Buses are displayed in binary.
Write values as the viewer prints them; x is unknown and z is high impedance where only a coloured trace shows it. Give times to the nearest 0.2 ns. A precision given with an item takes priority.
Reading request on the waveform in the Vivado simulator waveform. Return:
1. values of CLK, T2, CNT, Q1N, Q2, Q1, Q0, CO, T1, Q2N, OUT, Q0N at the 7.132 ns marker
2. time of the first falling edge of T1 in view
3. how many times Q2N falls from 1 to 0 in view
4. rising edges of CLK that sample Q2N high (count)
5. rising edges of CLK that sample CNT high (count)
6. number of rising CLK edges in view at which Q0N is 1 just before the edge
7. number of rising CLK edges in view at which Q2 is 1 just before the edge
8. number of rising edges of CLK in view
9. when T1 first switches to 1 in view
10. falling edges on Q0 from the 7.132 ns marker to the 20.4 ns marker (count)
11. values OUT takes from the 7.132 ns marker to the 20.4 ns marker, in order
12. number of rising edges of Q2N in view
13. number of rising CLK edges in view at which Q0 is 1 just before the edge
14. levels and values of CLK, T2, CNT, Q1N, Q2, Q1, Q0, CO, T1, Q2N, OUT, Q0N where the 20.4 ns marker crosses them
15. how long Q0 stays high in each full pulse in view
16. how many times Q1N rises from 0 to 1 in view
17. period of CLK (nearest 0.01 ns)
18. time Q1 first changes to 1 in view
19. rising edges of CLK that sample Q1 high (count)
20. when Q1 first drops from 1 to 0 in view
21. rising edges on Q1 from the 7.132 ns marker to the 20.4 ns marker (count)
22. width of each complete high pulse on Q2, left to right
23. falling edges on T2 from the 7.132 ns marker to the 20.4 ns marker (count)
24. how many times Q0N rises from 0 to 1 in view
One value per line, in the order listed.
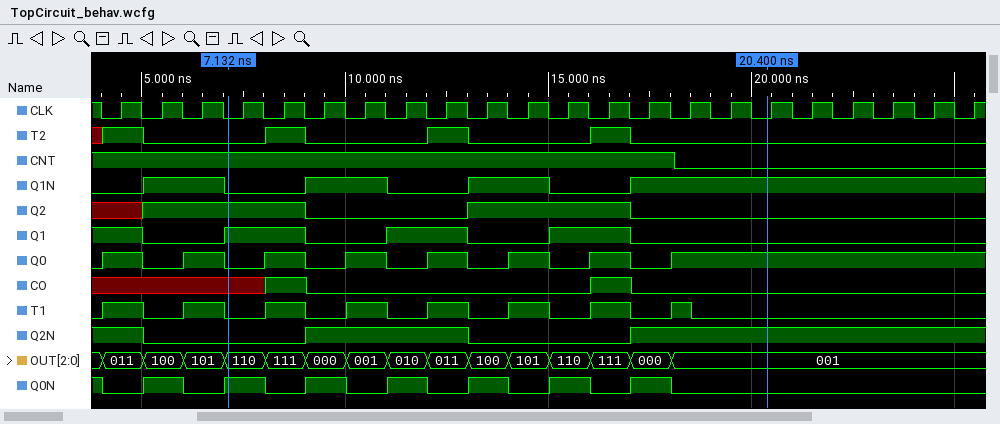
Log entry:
CLK=0, T2=0, CNT=1, Q1N=0, Q2=1, Q1=1, Q0=0, CO=x, T1=0, Q2N=0, OUT=110, Q0N=1
5 ns
2
14
14
7
8
22
4 ns
5
110, 111, 000, 001, 010, 011, 100, 101, 110, 111, 000, 001
2
15
CLK=0, T2=0, CNT=0, Q1N=1, Q2=0, Q1=0, Q0=1, CO=0, T1=0, Q2N=1, OUT=001, Q0N=0
1 ns, 1 ns, 1 ns, 1 ns, 1 ns, 1 ns, 1 ns
4
1 ns
7 ns
7
5 ns
2
4 ns
3
7
